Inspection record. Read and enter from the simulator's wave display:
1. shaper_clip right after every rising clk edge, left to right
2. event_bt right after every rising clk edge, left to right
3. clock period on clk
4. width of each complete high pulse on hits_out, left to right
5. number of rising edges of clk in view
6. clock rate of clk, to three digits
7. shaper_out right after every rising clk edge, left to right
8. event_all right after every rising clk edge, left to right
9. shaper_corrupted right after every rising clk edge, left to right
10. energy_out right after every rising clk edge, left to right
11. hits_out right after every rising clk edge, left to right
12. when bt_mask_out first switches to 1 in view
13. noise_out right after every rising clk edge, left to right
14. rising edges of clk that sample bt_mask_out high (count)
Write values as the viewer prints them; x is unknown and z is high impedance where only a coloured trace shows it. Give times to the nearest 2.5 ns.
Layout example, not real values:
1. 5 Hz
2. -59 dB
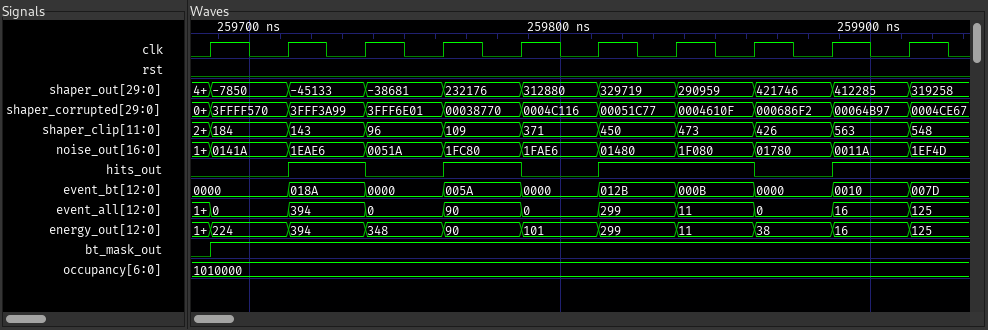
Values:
1. 184, 143, 96, 109, 371, 450, 473, 426, 563, 548
2. 0000, 018A, 0000, 005A, 0000, 012B, 000B, 0000, 0010, 007D
3. 25 ns
4. 25 ns, 25 ns, 50 ns
5. 10
6. 40.0 MHz
7. -7850, -45133, -38681, 232176, 312880, 329719, 290959, 421746, 412285, 319258
8. 0, 394, 0, 90, 0, 299, 11, 0, 16, 125
9. 3FFFF570, 3FFF3A99, 3FFF6E01, 00038770, 0004C116, 00051C77, 0004610F, 000686F2, 00064B97, 0004CE67
10. 224, 394, 348, 90, 101, 299, 11, 38, 16, 125
11. 0 1 0 1 0 1 1 0 1 1
12. 259687.5 ns
13. 0141A, 1EAE6, 0051A, 1FC80, 1FAE6, 01480, 1F080, 01780, 0011A, 1EF4D
14. 9
